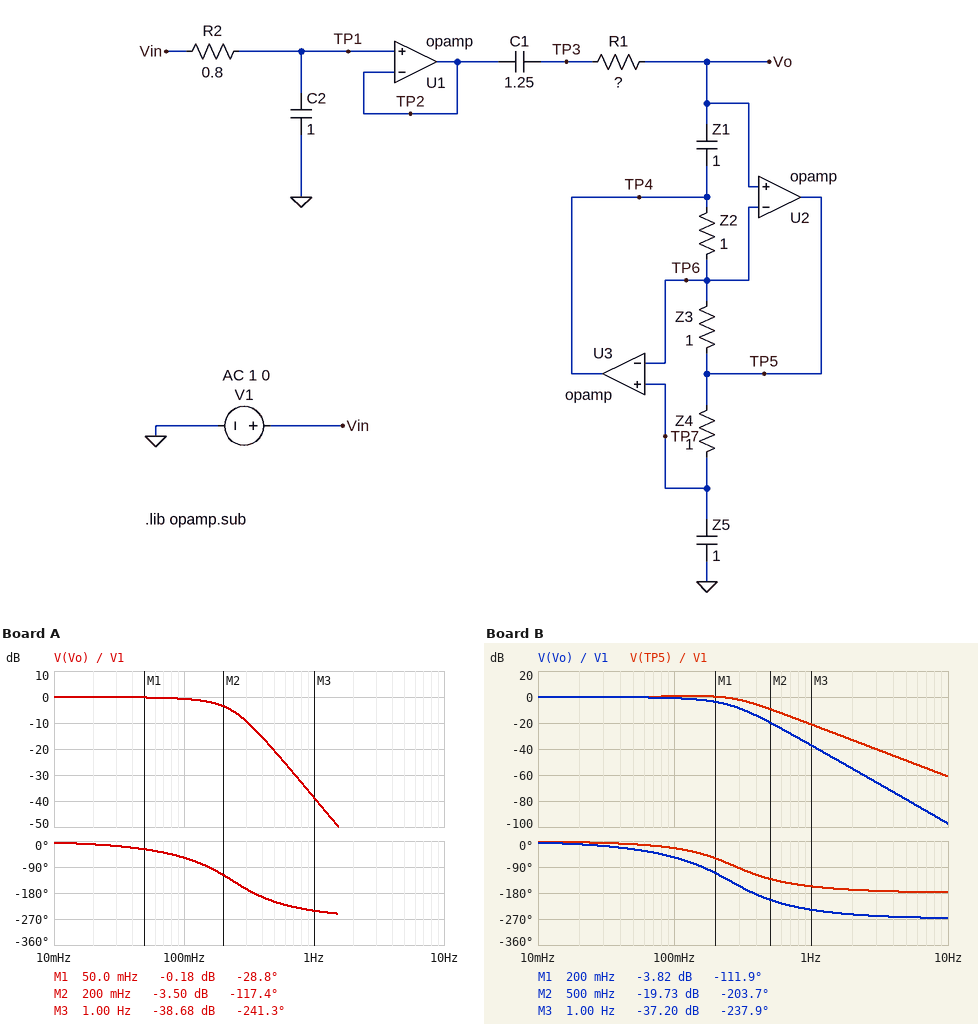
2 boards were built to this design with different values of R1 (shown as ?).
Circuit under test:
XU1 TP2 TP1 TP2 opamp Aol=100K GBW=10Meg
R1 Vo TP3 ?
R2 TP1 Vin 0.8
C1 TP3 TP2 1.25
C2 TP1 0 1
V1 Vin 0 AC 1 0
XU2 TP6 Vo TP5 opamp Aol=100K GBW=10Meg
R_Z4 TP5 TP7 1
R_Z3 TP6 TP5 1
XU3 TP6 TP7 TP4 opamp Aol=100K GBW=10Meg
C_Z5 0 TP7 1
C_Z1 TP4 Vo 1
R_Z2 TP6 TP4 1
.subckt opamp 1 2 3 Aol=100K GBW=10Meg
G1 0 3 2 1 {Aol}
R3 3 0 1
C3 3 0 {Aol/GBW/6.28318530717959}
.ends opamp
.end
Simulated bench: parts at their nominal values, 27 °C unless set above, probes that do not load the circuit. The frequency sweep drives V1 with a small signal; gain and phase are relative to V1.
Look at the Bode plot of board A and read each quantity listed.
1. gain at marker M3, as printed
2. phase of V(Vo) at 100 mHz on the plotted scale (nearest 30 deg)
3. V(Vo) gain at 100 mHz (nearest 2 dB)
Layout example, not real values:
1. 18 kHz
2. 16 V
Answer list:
1. -38.68 dB
2. -60 deg
3. 0 dB
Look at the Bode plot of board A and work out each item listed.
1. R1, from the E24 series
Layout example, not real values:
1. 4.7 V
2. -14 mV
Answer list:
1. 0.43 Ω
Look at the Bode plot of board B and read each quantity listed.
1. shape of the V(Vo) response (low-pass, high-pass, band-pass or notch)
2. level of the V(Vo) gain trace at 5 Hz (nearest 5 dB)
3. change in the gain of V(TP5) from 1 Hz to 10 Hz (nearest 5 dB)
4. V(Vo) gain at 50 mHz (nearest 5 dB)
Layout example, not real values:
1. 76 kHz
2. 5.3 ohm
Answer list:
1. low-pass
2. -80 dB
3. -40 dB
4. 0 dB
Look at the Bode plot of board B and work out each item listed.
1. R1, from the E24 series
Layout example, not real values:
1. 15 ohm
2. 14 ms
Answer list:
1. 0.36 Ω
